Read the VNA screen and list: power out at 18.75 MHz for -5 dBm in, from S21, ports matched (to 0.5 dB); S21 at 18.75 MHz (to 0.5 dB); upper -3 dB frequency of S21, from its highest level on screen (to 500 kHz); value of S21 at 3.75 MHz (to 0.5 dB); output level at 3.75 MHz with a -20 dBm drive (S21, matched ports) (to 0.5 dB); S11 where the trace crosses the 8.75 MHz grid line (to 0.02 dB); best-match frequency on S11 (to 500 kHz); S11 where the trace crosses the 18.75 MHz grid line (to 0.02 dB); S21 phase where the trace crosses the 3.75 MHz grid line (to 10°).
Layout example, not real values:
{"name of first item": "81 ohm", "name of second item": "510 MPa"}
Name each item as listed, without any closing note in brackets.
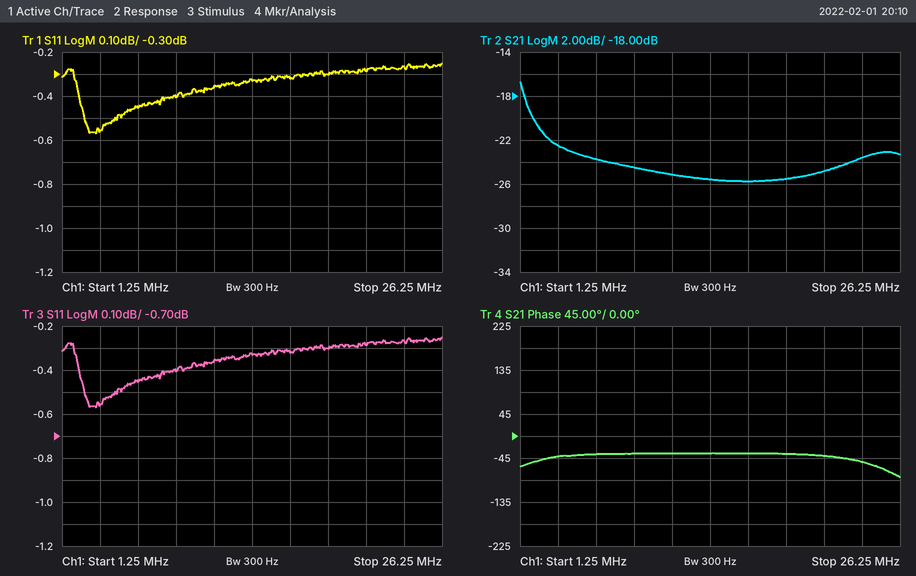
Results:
{"power out at 18.75 MHz for -5 dBm in, from S21, ports matched": "-30.5 dBm", "S21 at 18.75 MHz": "-25.5 dB", "upper -3 dB frequency of S21, from its highest level on screen": "2.0 MHz", "value of S21 at 3.75 MHz": "-22.5 dB", "output level at 3.75 MHz with a -20 dBm drive (S21, matched ports)": "-42.5 dBm", "S11 where the trace crosses the 8.75 MHz grid line": "-0.40 dB", "best-match frequency on S11": "3.5 MHz", "S11 where the trace crosses the 18.75 MHz grid line": "-0.30 dB", "S21 phase where the trace crosses the 3.75 MHz grid line": "-40°"}
